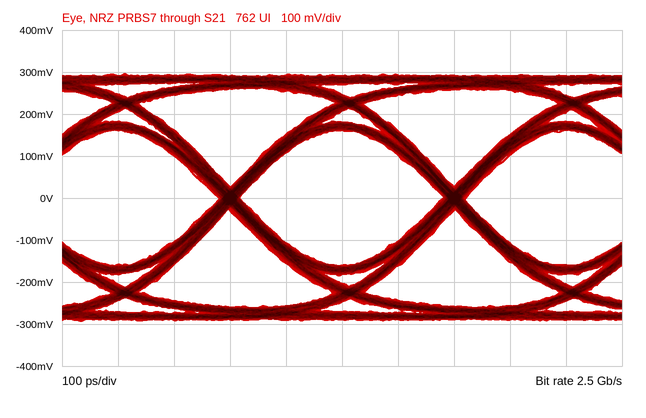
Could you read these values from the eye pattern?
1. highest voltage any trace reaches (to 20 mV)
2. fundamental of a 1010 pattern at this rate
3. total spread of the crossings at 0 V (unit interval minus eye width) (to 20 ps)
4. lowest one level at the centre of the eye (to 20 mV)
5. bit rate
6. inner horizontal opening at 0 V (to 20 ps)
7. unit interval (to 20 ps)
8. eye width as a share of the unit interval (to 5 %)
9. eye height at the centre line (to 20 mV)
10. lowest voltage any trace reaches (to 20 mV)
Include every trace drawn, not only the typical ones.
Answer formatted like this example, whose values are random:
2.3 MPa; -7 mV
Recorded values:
300 mV; 1.25 GHz; 40 ps; 160 mV; 2.5 Gb/s; 360 ps; 400 ps; 90 %; 320 mV; -300 mV
